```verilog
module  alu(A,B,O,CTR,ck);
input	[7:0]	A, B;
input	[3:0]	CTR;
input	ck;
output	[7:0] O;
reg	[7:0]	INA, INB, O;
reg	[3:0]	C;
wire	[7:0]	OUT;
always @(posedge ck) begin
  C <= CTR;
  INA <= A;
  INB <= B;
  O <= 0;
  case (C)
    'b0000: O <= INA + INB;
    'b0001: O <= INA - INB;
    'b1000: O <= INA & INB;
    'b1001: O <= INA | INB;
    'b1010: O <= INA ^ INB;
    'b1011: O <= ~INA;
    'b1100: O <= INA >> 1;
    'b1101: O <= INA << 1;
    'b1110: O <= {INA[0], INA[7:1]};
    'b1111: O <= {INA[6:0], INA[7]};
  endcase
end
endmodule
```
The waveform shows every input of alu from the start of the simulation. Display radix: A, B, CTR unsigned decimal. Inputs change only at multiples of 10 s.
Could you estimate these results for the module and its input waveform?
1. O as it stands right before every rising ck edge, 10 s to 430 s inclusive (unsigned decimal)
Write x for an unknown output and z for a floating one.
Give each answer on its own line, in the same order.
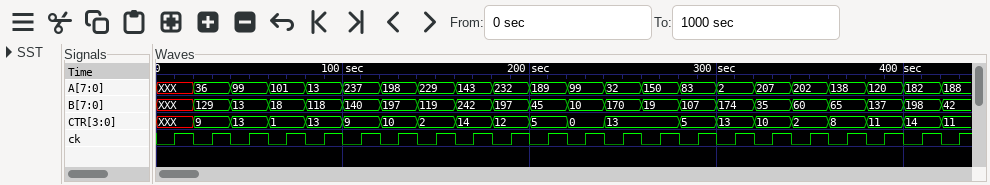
x, 0, 0, 165, 198, 83, 26, 237, 3, 0, 199, 116, 0, 109, 64, 44, 0, 4, 236, 0, 0, 135
